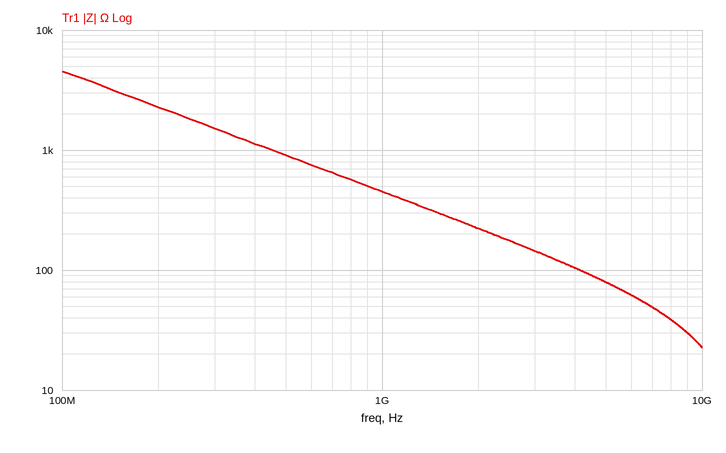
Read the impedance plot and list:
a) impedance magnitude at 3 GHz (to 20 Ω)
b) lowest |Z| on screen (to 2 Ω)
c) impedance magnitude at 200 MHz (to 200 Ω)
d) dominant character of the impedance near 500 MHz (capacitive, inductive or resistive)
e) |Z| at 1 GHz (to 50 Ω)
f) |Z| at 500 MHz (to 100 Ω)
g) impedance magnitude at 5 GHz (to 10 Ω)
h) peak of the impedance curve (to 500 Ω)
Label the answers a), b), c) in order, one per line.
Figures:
a) 140 Ω
b) 22 Ω
c) 2.2 kΩ
d) capacitive
e) 450 Ω
f) 900 Ω
g) 80 Ω
h) 4.5 kΩ
